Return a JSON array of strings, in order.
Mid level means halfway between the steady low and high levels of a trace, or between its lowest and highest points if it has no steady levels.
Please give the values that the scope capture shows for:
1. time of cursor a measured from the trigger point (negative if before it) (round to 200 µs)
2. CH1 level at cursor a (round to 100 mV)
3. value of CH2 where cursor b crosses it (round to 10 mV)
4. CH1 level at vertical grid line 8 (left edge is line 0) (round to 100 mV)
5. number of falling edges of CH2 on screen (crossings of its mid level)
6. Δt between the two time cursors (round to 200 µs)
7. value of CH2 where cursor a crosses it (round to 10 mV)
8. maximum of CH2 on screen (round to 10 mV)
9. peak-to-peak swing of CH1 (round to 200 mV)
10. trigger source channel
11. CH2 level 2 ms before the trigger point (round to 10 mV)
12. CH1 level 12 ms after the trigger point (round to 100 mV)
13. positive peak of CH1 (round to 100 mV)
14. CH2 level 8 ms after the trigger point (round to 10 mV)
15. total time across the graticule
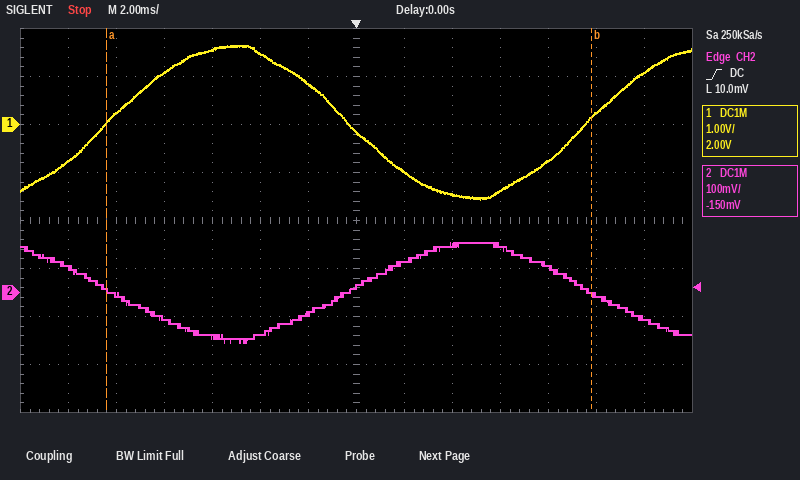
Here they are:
["-10.4 ms", "0.0 V", "0 mV", "-1.0 V", "2", "20.2 ms", "10 mV", "100 mV", "3.2 V", "CH2", "-40 mV", "1.1 V", "1.6 V", "50 mV", "28 ms"]
